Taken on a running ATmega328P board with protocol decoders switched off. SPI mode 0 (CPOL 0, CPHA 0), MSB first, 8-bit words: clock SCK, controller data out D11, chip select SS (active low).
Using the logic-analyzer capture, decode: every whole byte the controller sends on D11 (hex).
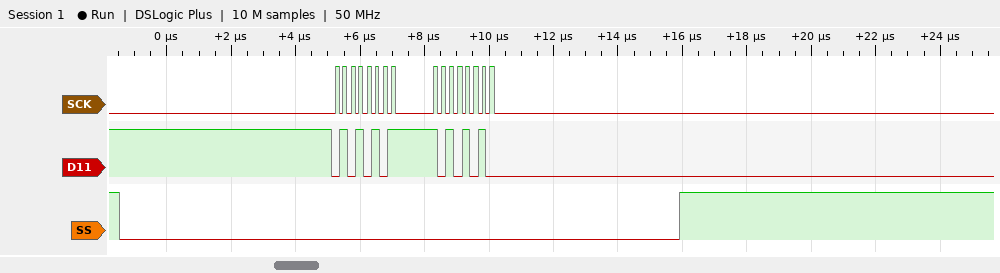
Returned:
0x55 0xAA
